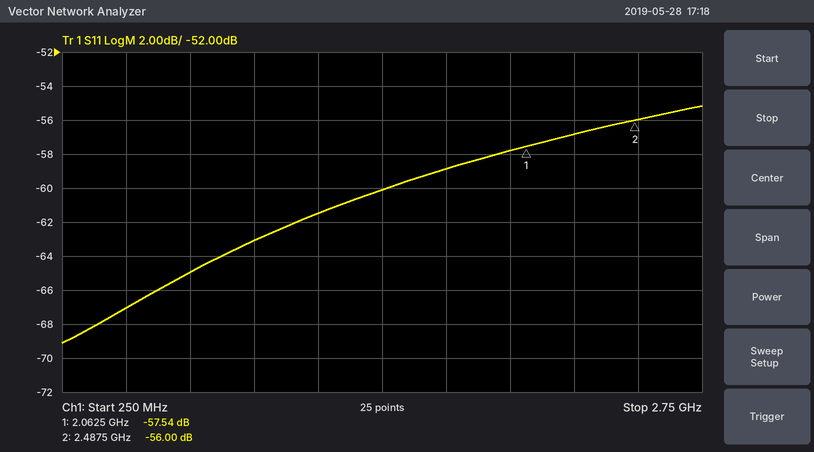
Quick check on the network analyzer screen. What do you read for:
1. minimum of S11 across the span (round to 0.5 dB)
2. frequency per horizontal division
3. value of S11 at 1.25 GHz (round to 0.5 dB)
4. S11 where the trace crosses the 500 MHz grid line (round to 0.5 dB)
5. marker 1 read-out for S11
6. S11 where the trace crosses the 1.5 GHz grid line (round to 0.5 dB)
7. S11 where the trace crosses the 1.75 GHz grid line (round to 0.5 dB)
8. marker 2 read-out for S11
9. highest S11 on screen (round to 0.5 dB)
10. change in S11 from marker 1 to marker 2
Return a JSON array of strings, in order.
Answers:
["-69.0 dB", "250 MHz", "-61.5 dB", "-67.0 dB", "-57.54 dB", "-60.0 dB", "-59.0 dB", "-56.00 dB", "-55.0 dB", "1.54 dB"]
